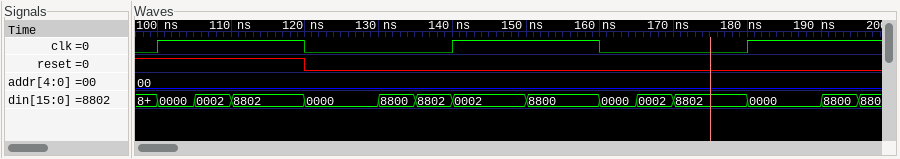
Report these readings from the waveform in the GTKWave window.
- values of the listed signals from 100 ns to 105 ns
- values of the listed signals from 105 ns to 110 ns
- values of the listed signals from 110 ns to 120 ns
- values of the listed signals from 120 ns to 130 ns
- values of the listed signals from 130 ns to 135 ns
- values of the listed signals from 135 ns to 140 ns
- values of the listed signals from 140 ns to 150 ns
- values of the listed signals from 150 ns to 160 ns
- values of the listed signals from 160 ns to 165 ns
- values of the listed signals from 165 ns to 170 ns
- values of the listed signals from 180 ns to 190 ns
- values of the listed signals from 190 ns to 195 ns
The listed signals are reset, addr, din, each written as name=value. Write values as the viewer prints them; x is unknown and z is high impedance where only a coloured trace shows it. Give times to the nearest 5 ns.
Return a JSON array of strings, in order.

["reset=1, addr=00, din=0000", "reset=1, addr=00, din=0002", "reset=1, addr=00, din=8802", "reset=0, addr=00, din=0000", "reset=0, addr=00, din=8800", "reset=0, addr=00, din=8802", "reset=0, addr=00, din=0002", "reset=0, addr=00, din=8800", "reset=0, addr=00, din=0000", "reset=0, addr=00, din=0002", "reset=0, addr=00, din=0000", "reset=0, addr=00, din=8800"]
